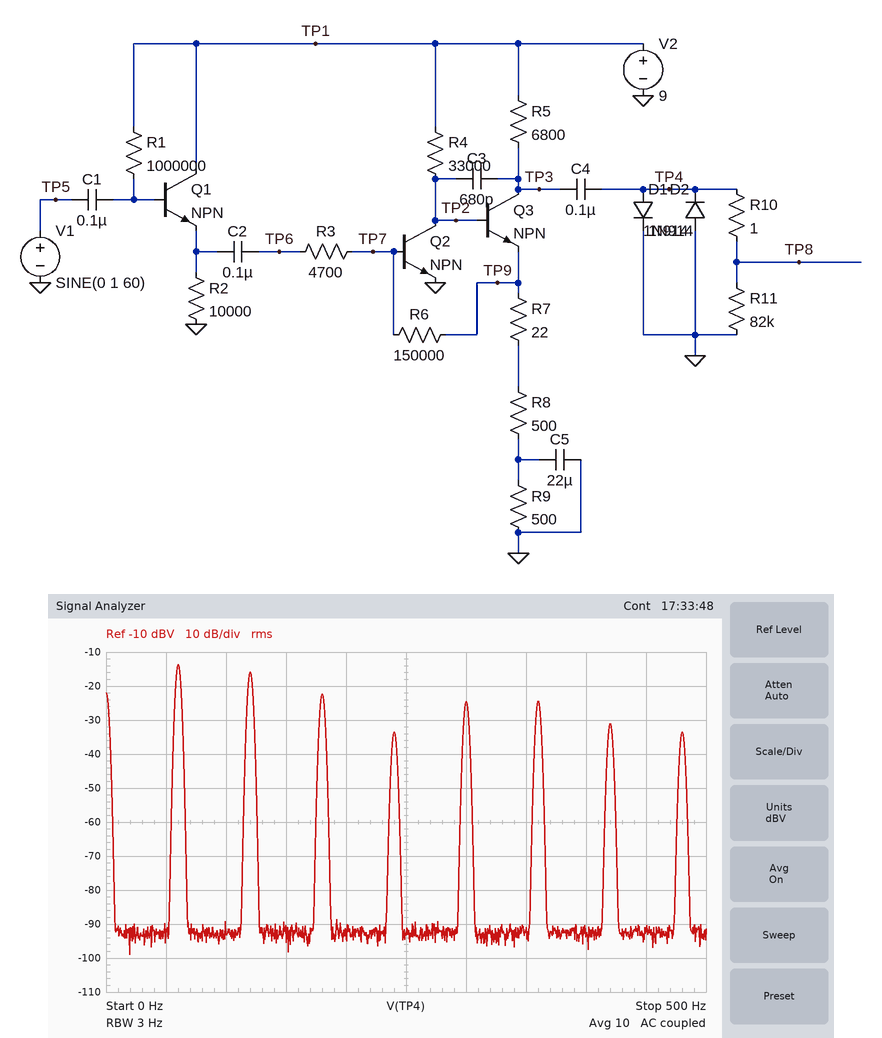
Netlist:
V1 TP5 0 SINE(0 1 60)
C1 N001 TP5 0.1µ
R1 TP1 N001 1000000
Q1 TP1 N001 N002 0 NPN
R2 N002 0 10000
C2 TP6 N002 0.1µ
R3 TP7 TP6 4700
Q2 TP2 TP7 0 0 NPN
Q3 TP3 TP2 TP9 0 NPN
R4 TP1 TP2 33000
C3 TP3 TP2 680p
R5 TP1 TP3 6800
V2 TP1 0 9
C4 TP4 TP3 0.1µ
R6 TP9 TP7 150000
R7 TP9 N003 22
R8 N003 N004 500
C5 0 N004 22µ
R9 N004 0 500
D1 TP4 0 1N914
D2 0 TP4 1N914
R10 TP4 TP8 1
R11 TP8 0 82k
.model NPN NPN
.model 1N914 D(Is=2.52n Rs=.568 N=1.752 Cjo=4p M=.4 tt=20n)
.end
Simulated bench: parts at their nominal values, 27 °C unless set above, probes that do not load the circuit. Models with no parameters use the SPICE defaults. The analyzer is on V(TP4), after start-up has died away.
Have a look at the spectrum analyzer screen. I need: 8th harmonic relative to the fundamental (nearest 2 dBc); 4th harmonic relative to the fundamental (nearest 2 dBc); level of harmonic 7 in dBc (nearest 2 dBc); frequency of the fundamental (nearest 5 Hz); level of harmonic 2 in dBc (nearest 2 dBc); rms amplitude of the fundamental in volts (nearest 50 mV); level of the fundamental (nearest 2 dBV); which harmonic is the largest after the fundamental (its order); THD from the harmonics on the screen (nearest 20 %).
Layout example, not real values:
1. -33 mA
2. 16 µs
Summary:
1. -20 dBc
2. -20 dBc
3. -18 dBc
4. 60 Hz
5. -2 dBc
6. 200 mV
7. -14 dBV
8. 2
9. 100 %
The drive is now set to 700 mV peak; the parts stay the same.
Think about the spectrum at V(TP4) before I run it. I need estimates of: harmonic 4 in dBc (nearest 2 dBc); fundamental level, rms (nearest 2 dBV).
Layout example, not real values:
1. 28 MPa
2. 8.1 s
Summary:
1. -18 dBc
2. -14 dBV
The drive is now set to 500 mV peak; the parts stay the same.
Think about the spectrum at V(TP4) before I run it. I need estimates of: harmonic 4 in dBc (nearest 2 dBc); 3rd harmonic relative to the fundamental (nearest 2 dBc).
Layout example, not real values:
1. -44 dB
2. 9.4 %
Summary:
1. -16 dBc
2. -10 dBc
